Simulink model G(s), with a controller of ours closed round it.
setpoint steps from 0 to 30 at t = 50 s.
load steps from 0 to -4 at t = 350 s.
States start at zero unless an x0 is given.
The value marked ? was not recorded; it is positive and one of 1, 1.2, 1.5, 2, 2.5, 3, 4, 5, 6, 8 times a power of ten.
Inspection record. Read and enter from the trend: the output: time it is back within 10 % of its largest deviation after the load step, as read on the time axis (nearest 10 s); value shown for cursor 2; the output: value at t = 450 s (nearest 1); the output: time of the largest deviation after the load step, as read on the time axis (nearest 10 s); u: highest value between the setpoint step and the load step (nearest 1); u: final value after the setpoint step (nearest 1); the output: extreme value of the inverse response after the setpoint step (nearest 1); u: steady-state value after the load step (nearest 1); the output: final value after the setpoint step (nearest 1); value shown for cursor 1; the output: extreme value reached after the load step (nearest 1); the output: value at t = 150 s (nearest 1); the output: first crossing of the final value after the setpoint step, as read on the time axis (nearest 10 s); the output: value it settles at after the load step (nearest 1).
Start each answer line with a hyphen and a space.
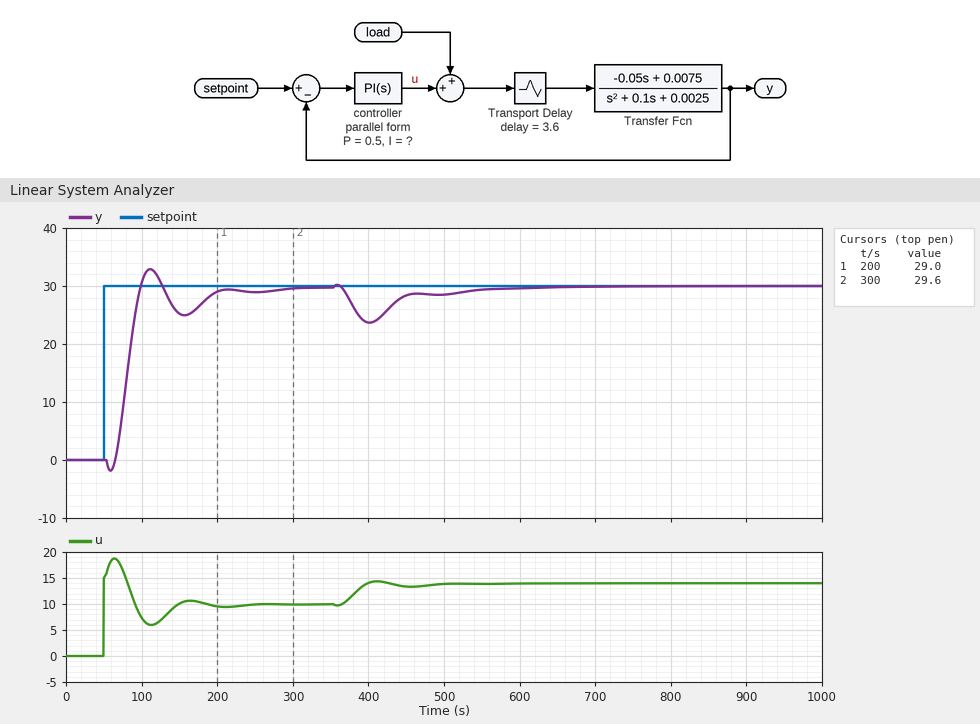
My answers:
- 550 s
- 29.6
- 28
- 400 s
- 19
- 10
- -2
- 14
- 30
- 29.0
- 24
- 25
- 100 s
- 30
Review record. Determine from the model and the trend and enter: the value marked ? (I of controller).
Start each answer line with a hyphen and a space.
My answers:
- 0.008
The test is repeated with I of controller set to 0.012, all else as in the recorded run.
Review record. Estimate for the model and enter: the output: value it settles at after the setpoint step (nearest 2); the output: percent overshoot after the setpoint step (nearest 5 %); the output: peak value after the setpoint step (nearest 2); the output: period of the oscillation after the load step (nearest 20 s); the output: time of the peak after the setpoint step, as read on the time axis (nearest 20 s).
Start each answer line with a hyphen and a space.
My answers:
- 30
- 25 %
- 38
- 100 s
- 120 s
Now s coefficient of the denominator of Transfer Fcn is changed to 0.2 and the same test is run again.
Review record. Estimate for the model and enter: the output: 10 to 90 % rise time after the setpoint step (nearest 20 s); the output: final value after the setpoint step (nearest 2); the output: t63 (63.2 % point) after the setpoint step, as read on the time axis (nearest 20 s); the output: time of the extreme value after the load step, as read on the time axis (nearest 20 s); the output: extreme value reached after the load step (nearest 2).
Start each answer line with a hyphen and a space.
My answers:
- 60 s
- 30
- 100 s
- 420 s
- 26
